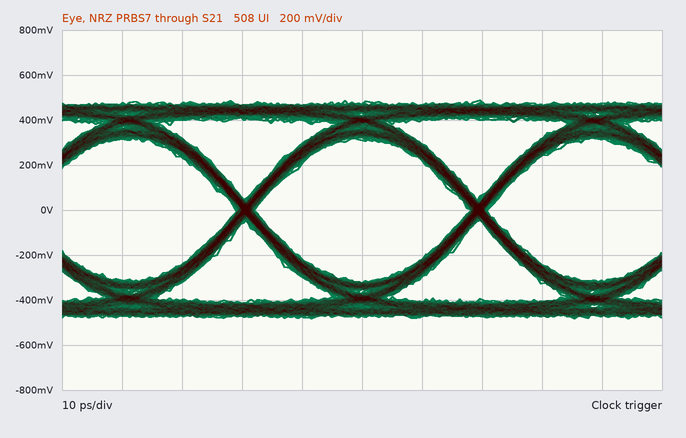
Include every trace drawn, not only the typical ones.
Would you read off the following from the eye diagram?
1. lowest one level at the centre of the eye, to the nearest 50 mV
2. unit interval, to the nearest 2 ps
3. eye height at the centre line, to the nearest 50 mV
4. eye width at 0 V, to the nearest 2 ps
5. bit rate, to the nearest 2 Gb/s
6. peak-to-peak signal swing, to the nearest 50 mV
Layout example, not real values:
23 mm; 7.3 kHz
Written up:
300 mV; 38 ps; 650 mV; 36 ps; 26 Gb/s; 950 mV
